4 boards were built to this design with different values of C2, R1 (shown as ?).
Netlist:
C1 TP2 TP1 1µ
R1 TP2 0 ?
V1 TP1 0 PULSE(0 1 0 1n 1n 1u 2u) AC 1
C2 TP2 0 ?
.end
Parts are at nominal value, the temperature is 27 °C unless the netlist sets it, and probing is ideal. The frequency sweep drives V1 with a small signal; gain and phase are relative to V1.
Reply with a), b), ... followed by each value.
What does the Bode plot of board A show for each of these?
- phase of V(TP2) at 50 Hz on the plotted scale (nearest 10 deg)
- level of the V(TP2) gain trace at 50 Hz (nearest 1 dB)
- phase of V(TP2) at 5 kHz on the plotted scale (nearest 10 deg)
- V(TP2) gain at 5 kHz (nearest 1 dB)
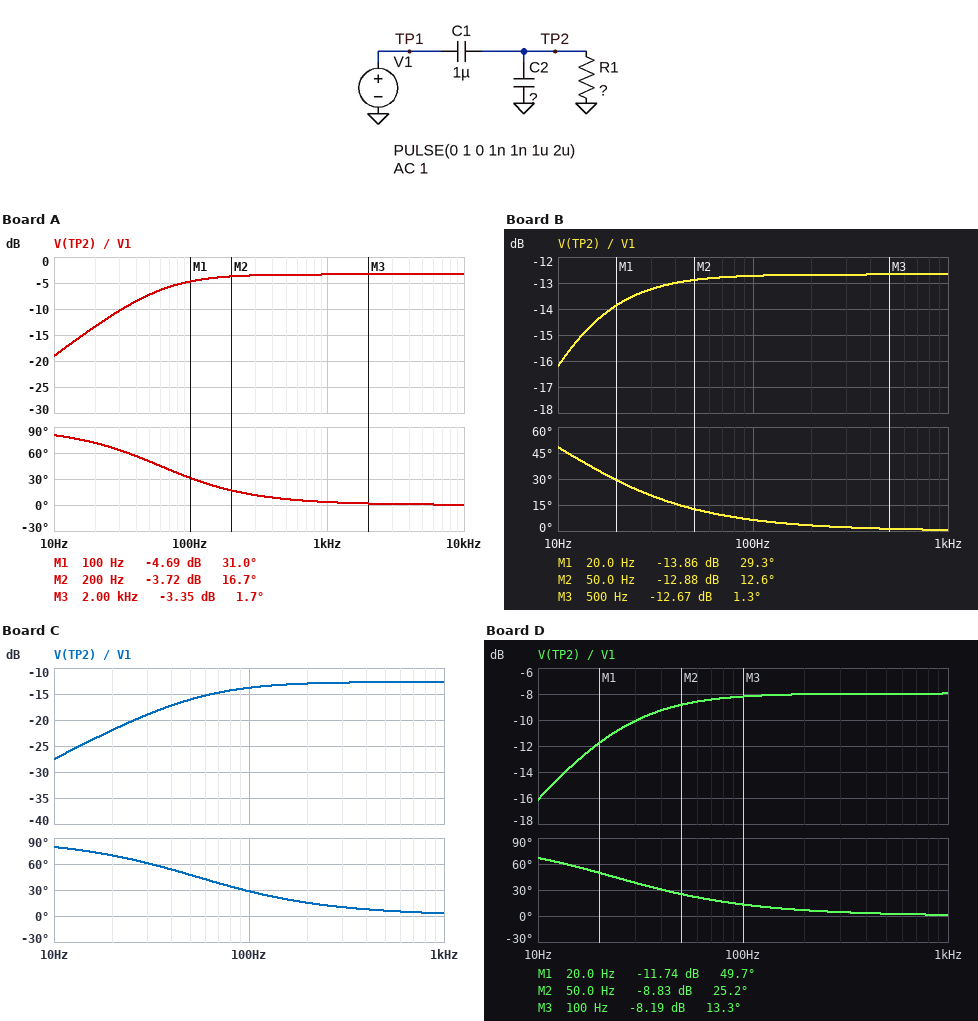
a) 50 deg
b) -7 dB
c) 0 deg
d) -3 dB
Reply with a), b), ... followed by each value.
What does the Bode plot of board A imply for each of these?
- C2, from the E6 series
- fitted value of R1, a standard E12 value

a) 470 nF
b) 1.8 kΩ
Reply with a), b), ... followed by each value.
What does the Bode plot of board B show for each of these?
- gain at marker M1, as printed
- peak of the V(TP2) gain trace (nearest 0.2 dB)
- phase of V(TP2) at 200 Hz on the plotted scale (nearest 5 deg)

a) -13.86 dB
b) -12.6 dB
c) 5 deg
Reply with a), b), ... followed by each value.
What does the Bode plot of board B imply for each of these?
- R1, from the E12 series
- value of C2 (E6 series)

a) 3.3 kΩ
b) 3.3 µF
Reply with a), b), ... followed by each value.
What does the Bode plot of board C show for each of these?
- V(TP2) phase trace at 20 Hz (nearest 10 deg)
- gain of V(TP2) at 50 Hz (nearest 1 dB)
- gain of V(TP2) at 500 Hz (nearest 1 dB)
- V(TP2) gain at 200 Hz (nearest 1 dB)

a) 70 deg
b) -16 dB
c) -13 dB
d) -13 dB
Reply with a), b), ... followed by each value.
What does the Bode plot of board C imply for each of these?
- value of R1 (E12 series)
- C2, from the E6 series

a) 680 Ω
b) 3.3 µF
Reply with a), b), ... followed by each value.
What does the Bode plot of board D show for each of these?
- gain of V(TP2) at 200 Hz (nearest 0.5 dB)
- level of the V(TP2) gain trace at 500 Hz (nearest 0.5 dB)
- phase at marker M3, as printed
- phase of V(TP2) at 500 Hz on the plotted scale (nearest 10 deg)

a) -8.0 dB
b) -8.0 dB
c) 13.3 deg
d) 0 deg
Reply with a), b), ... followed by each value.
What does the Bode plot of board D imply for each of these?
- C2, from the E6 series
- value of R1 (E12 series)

a) 1.5 µF
b) 2.7 kΩ
